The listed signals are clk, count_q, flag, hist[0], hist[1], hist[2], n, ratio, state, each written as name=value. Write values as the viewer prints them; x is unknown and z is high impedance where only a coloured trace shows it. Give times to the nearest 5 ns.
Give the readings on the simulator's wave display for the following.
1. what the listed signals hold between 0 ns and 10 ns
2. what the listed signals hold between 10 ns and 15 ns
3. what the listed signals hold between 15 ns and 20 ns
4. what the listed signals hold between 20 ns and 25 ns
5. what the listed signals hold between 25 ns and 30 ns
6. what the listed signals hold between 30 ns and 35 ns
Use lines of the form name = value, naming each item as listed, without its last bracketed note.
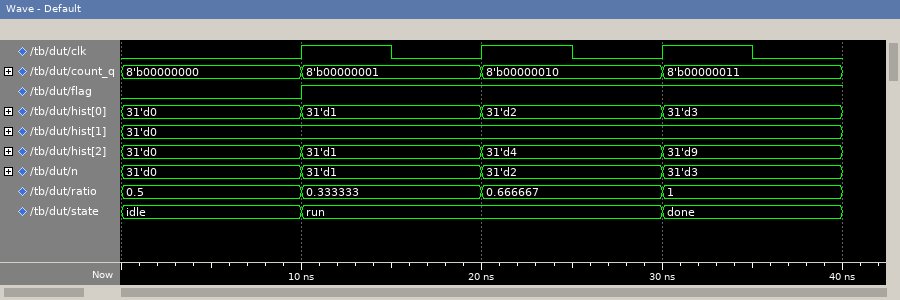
what the listed signals hold between 0 ns and 10 ns = clk=0, count_q=8'b00000000, flag=0, hist[0]=31'd0, hist[1]=31'd0, hist[2]=31'd0, n=31'd0, ratio=0.5, state=idle
what the listed signals hold between 10 ns and 15 ns = clk=1, count_q=8'b00000001, flag=1, hist[0]=31'd1, hist[1]=31'd0, hist[2]=31'd1, n=31'd1, ratio=0.333333, state=run
what the listed signals hold between 15 ns and 20 ns = clk=0, count_q=8'b00000001, flag=1, hist[0]=31'd1, hist[1]=31'd0, hist[2]=31'd1, n=31'd1, ratio=0.333333, state=run
what the listed signals hold between 20 ns and 25 ns = clk=1, count_q=8'b00000010, flag=1, hist[0]=31'd2, hist[1]=31'd0, hist[2]=31'd4, n=31'd2, ratio=0.666667, state=run
what the listed signals hold between 25 ns and 30 ns = clk=0, count_q=8'b00000010, flag=1, hist[0]=31'd2, hist[1]=31'd0, hist[2]=31'd4, n=31'd2, ratio=0.666667, state=run
what the listed signals hold between 30 ns and 35 ns = clk=1, count_q=8'b00000011, flag=1, hist[0]=31'd3, hist[1]=31'd0, hist[2]=31'd9, n=31'd3, ratio=1, state=done
